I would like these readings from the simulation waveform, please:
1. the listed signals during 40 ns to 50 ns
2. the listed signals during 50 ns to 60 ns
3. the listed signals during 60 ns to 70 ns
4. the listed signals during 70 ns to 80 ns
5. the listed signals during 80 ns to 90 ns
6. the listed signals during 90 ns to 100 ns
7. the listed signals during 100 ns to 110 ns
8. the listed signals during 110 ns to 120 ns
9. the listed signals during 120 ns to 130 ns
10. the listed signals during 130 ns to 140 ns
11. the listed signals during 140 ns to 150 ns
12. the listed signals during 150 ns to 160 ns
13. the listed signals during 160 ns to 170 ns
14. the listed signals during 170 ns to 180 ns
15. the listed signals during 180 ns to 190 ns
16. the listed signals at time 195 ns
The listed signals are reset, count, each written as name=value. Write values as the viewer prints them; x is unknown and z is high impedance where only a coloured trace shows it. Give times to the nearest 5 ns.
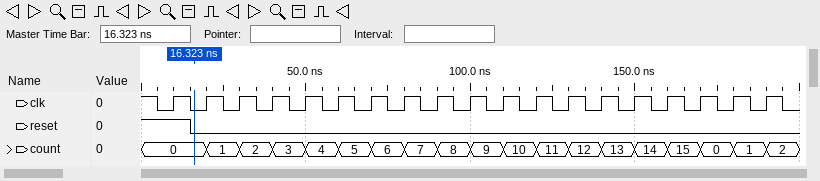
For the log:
reset=0, count=3
reset=0, count=4
reset=0, count=5
reset=0, count=6
reset=0, count=7
reset=0, count=8
reset=0, count=9
reset=0, count=10
reset=0, count=11
reset=0, count=12
reset=0, count=13
reset=0, count=14
reset=0, count=15
reset=0, count=0
reset=0, count=1
reset=0, count=2
